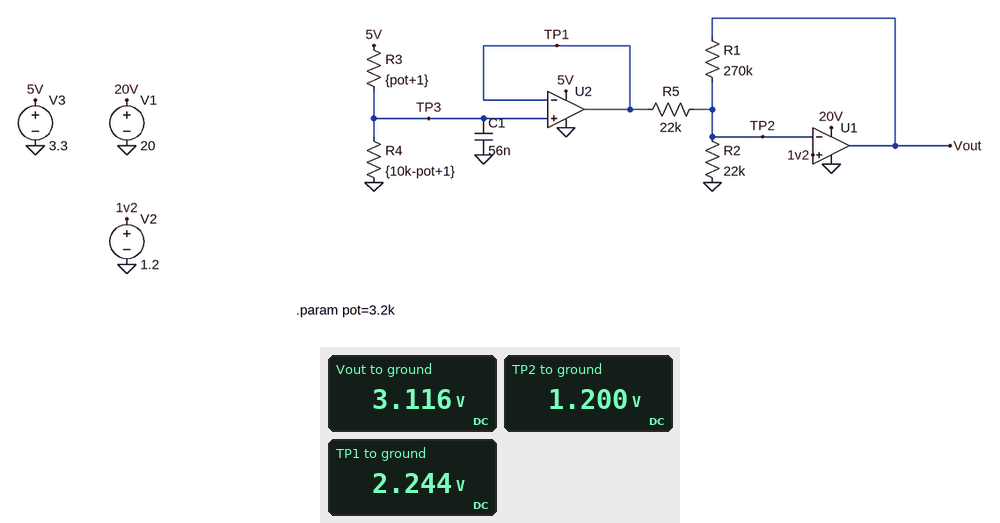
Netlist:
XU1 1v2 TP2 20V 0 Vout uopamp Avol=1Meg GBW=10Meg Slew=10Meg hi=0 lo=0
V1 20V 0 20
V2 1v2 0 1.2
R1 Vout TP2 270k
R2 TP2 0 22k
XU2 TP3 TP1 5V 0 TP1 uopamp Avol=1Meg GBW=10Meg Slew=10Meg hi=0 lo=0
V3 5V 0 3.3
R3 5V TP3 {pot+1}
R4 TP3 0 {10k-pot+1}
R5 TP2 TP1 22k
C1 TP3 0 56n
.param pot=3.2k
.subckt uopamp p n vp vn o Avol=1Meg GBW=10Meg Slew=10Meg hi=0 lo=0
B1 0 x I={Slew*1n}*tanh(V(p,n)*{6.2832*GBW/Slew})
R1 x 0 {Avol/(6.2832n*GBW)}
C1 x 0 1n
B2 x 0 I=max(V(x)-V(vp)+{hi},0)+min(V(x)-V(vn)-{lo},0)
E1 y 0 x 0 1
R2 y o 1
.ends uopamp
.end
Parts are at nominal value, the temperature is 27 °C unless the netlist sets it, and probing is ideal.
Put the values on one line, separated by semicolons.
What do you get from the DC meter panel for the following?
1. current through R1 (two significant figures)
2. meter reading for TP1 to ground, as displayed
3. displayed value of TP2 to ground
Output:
7.1 µA; 2.244 V; 1.200 V
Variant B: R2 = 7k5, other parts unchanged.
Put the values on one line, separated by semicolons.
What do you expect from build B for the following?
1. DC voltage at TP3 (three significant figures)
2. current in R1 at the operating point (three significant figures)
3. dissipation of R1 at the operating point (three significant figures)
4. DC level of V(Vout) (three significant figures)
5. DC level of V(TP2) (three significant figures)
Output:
2.24 V; 70.5 µA; 1.34 mW; 20.0 V; 965 mV
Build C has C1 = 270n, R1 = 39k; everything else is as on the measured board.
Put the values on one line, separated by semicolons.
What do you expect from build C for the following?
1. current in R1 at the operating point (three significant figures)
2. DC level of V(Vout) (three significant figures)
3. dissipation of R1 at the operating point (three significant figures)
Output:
7.10 µA; 1.48 V; 1.96 µW
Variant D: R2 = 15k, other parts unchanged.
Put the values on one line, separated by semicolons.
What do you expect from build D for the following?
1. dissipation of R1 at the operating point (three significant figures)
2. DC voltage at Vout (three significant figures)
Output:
286 µW; 9.99 V
